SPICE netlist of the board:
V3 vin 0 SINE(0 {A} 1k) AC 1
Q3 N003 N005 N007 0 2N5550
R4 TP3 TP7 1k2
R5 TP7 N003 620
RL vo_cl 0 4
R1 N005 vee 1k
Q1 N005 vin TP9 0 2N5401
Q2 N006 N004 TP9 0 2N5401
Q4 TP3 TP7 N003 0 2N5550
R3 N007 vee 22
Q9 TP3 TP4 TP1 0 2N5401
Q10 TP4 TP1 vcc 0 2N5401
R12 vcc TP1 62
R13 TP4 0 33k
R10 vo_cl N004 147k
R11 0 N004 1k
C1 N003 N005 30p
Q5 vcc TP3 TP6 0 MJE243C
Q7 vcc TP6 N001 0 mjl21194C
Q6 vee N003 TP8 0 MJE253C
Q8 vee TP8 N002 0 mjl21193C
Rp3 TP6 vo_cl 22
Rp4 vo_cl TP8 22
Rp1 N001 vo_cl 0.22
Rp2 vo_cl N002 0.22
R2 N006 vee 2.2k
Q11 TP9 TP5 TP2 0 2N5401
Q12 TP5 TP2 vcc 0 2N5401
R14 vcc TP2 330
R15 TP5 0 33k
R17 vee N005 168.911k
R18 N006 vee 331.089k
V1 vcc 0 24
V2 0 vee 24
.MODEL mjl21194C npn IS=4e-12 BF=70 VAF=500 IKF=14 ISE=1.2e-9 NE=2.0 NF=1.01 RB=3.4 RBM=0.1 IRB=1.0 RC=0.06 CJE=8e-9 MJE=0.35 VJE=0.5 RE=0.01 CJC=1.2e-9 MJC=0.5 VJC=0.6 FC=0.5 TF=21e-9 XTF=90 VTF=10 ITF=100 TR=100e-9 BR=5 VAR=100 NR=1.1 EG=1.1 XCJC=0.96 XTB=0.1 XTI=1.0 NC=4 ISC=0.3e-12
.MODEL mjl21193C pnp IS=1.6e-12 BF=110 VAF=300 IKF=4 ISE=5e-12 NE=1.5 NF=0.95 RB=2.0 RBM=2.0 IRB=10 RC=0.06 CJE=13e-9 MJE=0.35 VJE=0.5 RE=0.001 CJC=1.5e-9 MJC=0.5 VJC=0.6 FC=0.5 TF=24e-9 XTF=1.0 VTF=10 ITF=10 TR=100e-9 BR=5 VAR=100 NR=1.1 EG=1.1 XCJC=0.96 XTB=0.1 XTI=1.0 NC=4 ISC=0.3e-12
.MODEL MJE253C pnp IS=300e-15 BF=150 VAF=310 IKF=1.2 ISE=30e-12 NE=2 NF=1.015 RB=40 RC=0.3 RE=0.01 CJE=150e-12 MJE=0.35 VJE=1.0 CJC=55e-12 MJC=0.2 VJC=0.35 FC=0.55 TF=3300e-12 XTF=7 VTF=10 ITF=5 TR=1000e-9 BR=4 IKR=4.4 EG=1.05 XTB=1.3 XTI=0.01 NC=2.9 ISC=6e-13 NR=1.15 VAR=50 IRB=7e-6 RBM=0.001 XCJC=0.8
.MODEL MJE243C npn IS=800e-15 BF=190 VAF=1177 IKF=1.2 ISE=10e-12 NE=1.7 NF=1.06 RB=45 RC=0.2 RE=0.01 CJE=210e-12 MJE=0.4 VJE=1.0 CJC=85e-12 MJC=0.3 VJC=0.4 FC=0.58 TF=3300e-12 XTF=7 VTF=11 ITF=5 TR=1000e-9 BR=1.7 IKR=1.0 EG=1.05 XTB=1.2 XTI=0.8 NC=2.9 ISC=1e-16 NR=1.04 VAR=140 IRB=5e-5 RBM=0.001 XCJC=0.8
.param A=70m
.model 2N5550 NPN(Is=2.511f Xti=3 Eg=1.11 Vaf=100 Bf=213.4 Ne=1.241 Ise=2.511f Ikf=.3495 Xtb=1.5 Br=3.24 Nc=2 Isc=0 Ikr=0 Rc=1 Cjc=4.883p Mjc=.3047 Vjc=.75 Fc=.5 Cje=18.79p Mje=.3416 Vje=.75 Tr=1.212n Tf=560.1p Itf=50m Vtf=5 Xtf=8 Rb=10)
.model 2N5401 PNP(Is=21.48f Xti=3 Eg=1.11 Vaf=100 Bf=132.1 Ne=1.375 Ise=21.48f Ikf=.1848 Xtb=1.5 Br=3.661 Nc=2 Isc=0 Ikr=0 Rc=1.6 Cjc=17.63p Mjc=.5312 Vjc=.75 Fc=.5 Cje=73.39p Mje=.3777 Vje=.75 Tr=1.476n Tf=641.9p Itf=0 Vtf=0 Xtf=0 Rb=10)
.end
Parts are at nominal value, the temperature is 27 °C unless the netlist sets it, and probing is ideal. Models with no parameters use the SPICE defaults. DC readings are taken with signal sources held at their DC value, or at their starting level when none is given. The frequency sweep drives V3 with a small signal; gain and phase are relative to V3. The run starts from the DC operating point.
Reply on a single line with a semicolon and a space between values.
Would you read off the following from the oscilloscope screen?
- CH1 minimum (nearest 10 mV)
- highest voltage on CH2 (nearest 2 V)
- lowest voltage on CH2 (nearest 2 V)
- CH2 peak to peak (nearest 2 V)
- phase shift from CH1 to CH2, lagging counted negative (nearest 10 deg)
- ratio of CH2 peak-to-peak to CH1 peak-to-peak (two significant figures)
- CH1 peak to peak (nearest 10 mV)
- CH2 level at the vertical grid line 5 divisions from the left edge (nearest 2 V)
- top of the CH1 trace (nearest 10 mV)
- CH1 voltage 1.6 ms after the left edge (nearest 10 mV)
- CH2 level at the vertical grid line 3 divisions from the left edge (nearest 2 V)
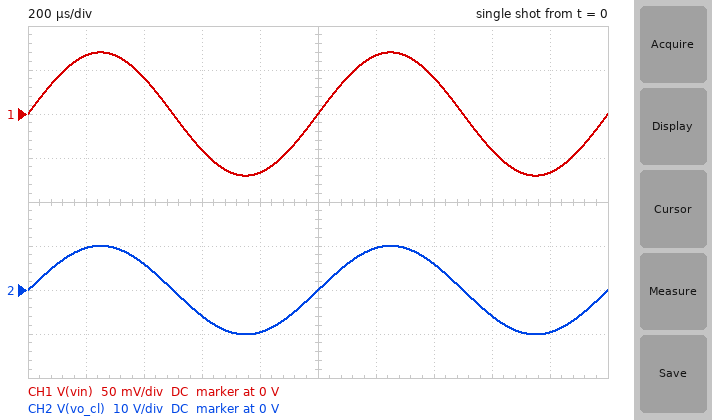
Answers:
-70 mV; 10 V; -10 V; 20 V; 0 deg; 140; 140 mV; 0 V; 70 mV; -40 mV; -6 V
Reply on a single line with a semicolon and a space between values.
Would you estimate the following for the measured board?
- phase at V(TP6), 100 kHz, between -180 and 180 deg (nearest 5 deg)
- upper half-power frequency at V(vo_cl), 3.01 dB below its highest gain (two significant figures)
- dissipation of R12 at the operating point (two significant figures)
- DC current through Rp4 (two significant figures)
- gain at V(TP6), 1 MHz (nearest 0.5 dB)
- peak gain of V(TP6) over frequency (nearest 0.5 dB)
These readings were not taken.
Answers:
-30 deg; 260 kHz; 6.3 mW; 24 mA; 31.5 dB; 48.0 dB
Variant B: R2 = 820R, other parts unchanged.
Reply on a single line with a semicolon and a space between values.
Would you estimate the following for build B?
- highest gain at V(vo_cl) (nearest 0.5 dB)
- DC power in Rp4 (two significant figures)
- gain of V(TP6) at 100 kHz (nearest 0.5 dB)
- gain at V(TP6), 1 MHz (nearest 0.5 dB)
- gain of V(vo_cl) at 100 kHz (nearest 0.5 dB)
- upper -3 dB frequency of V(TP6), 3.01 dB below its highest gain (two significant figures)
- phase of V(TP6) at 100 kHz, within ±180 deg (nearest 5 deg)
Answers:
40.5 dB; 10 mW; 48.5 dB; 32.5 dB; 39.5 dB; 160 kHz; -35 deg
